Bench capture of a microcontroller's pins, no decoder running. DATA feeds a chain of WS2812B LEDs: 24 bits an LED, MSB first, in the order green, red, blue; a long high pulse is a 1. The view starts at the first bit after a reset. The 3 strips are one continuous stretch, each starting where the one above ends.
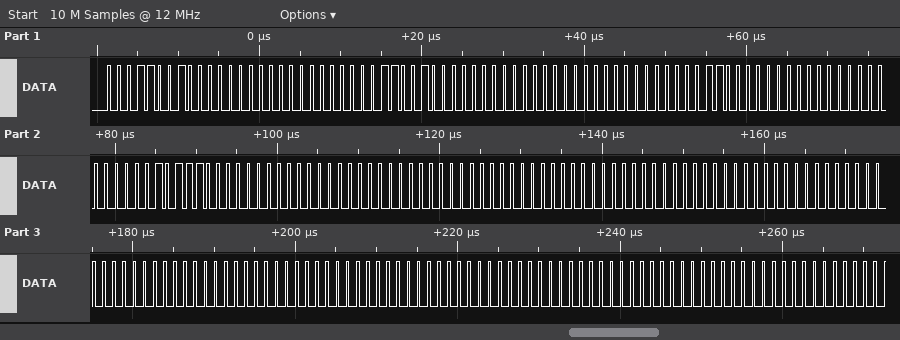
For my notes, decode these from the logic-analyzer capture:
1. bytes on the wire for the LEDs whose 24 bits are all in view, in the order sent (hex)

19 00 00 19 00 00 00 18 00 00 17 00 00 00 00 00 00 00 00 00 00 00 00 00 00 00 00
